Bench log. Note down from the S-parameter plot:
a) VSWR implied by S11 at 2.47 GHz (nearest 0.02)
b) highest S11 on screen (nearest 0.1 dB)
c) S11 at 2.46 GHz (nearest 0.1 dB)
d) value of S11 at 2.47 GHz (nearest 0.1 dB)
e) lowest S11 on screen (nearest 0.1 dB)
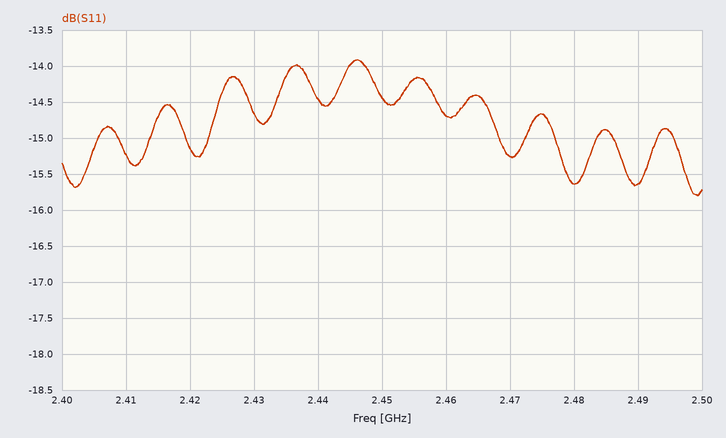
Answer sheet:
1.42
-13.9 dB
-14.7 dB
-15.3 dB
-15.8 dB
